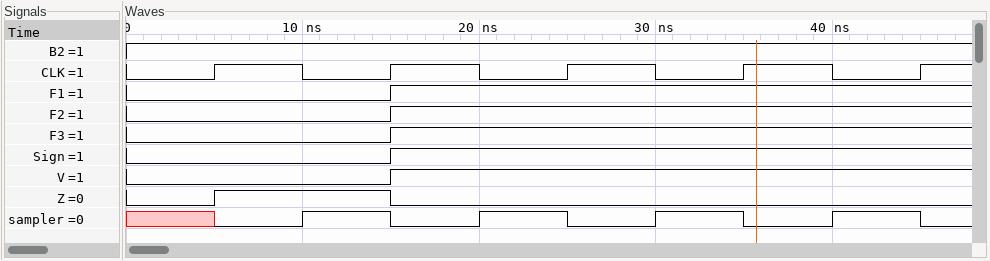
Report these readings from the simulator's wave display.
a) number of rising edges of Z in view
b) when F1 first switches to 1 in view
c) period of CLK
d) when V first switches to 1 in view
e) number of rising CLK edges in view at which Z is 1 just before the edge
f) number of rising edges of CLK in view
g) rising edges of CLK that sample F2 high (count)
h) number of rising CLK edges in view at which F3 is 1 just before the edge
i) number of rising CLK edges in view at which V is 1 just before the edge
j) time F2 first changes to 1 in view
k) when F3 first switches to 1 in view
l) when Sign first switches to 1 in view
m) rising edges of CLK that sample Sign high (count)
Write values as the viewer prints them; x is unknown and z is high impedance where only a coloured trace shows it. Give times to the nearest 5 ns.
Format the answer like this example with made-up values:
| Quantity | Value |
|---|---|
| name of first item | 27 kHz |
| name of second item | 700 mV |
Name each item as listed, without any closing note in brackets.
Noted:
| Quantity | Value |
|---|---|
| number of rising edges of Z in view | 1 |
| when F1 first switches to 1 in view | 15 ns |
| period of CLK | 10 ns |
| when V first switches to 1 in view | 15 ns |
| number of rising CLK edges in view at which Z is 1 just before the edge | 1 |
| number of rising edges of CLK in view | 5 |
| rising edges of CLK that sample F2 high | 3 |
| number of rising CLK edges in view at which F3 is 1 just before the edge | 3 |
| number of rising CLK edges in view at which V is 1 just before the edge | 3 |
| time F2 first changes to 1 in view | 15 ns |
| when F3 first switches to 1 in view | 15 ns |
| when Sign first switches to 1 in view | 15 ns |
| rising edges of CLK that sample Sign high | 3 |
